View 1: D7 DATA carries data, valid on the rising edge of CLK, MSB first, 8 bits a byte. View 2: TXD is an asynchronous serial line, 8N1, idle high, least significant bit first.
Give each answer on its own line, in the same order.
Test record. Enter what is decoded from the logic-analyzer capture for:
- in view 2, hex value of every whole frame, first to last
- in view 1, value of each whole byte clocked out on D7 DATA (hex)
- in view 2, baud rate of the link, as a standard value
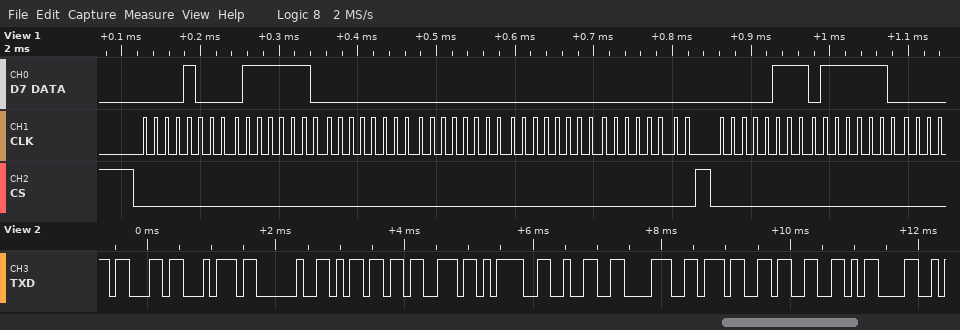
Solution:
63 74 20 6D 73 3D 32 38 37 33 0D
0x08 0x7E 0x00 0x00 0x00 0x00 0x07 0x7E
9600 baud
